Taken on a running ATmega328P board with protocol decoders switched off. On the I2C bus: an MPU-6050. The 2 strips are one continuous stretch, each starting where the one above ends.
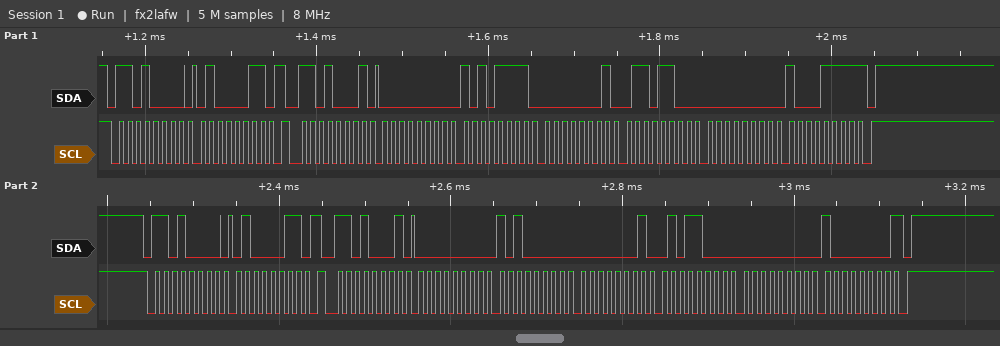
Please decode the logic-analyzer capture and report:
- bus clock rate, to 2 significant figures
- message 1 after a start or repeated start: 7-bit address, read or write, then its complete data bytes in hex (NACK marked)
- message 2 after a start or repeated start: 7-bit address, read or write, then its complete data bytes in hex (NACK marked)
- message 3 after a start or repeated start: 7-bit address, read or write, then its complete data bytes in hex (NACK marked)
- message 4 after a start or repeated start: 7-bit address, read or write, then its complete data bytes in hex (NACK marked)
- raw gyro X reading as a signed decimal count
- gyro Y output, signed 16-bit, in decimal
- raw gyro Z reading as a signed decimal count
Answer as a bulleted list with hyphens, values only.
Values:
- 100 kHz
- 0x68 write: 43
- 0x68 read: 00 AF 01 6C 00 8F NACK
- 0x68 write: 43
- 0x68 read: 00 A0 01 58 00 80 NACK
- 175
- 364
- 143
